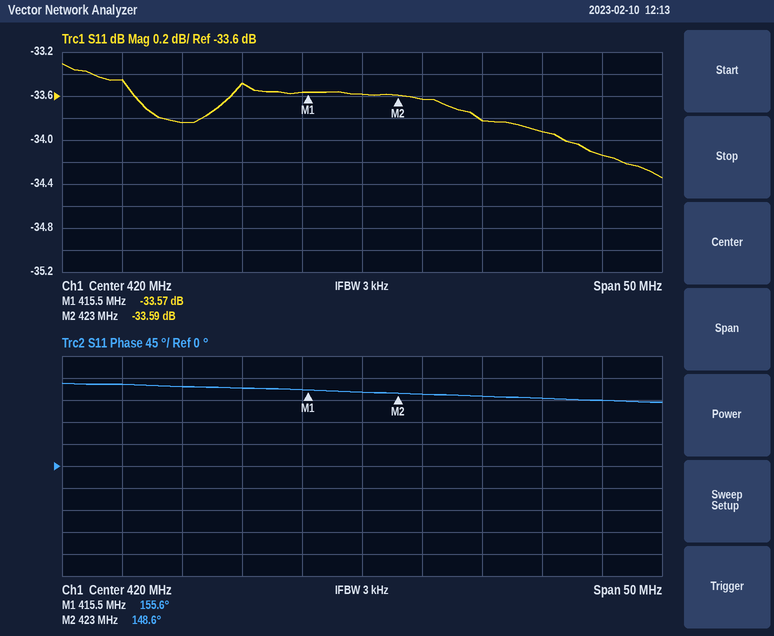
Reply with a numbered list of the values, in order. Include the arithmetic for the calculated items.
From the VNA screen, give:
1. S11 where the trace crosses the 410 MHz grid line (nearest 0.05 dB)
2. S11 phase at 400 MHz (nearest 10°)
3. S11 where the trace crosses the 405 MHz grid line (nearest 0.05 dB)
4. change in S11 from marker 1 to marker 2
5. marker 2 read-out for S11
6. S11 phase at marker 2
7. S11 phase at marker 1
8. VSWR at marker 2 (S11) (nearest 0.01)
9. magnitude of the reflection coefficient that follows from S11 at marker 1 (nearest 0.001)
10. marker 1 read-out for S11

1. -33.50 dB
2. 170°
3. -33.85 dB
4. -33.59 − (-33.57) = -0.02 dB
5. -33.59 dB
6. 148.6°
7. 155.6°
8. (1 + 0.0209)/(1 − 0.0209) ≈ 1.04
9. 10^(-33.57/20) ≈ 0.021
10. -33.57 dB
